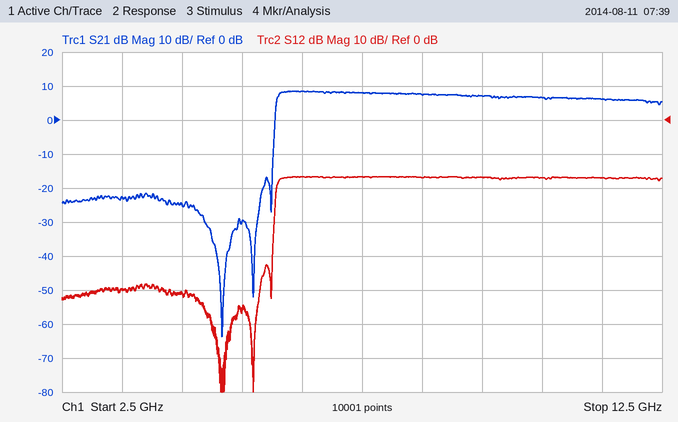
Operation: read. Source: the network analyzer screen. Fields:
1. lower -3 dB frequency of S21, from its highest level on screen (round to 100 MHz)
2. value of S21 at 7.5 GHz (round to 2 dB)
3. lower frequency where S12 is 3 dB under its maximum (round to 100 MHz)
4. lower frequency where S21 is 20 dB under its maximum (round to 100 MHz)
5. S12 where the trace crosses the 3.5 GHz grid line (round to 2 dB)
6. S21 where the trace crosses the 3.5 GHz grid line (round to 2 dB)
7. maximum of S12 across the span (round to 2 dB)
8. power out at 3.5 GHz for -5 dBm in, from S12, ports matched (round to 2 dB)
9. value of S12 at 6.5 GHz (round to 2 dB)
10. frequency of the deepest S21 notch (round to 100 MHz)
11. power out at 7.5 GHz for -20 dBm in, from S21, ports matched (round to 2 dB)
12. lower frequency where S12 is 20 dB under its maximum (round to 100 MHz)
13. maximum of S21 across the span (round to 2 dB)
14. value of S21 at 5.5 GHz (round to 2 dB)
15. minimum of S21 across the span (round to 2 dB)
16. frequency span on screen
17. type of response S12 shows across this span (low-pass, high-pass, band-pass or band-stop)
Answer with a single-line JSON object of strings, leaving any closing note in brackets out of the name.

{"lower -3 dB frequency of S21, from its highest level on screen": "6.1 GHz", "value of S21 at 7.5 GHz": "8 dB", "lower frequency where S12 is 3 dB under its maximum": "6.1 GHz", "lower frequency where S21 is 20 dB under its maximum": "6.0 GHz", "S12 where the trace crosses the 3.5 GHz grid line": "-50 dB", "S21 where the trace crosses the 3.5 GHz grid line": "-22 dB", "maximum of S12 across the span": "-16 dB", "power out at 3.5 GHz for -5 dBm in, from S12, ports matched": "-54 dBm", "value of S12 at 6.5 GHz": "-16 dB", "frequency of the deepest S21 notch": "5.2 GHz", "power out at 7.5 GHz for -20 dBm in, from S21, ports matched": "-12 dBm", "lower frequency where S12 is 20 dB under its maximum": "6.0 GHz", "maximum of S21 across the span": "8 dB", "value of S21 at 5.5 GHz": "-30 dB", "minimum of S21 across the span": "-64 dB", "frequency span on screen": "10 GHz", "type of response S12 shows across this span": "high-pass"}
